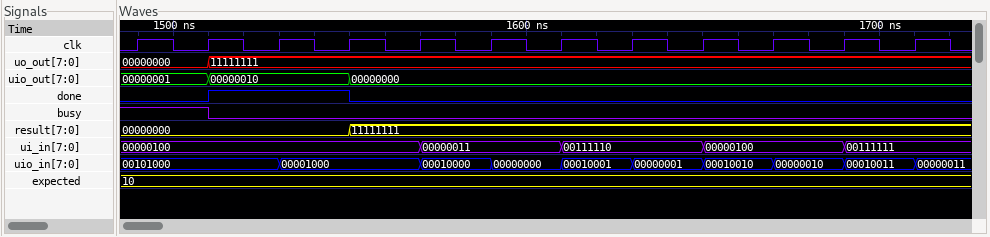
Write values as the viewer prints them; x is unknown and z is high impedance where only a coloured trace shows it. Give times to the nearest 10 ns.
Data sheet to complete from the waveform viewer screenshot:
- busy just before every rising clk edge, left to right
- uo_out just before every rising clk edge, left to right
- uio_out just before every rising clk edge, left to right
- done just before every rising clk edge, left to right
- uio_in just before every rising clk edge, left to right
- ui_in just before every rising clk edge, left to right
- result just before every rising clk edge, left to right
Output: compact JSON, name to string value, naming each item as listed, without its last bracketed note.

{"busy just before every rising clk edge, left to right": "1 1 0 0 0 0 0 0 0 0 0 0", "uo_out just before every rising clk edge, left to right": "00000000, 00000000, 11111111, 11111111, 11111111, 11111111, 11111111, 11111111, 11111111, 11111111, 11111111, 11111111", "uio_out just before every rising clk edge, left to right": "00000001, 00000001, 00000010, 00000010, 00000000, 00000000, 00000000, 00000000, 00000000, 00000000, 00000000, 00000000", "done just before every rising clk edge, left to right": "0 0 1 1 0 0 0 0 0 0 0 0", "uio_in just before every rising clk edge, left to right": "00101000, 00101000, 00101000, 00001000, 00001000, 00010000, 00000000, 00010001, 00000001, 00010010, 00000010, 00010011", "ui_in just before every rising clk edge, left to right": "00000100, 00000100, 00000100, 00000100, 00000100, 00000011, 00000011, 00111110, 00111110, 00000100, 00000100, 00111111", "result just before every rising clk edge, left to right": "00000000, 00000000, 00000000, 00000000, 11111111, 11111111, 11111111, 11111111, 11111111, 11111111, 11111111, 11111111"}
